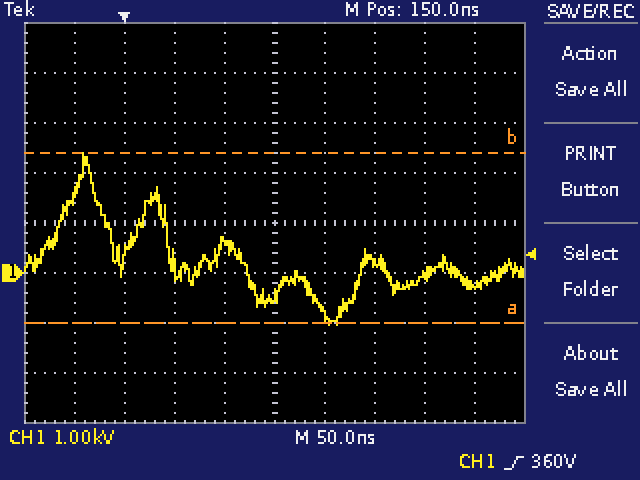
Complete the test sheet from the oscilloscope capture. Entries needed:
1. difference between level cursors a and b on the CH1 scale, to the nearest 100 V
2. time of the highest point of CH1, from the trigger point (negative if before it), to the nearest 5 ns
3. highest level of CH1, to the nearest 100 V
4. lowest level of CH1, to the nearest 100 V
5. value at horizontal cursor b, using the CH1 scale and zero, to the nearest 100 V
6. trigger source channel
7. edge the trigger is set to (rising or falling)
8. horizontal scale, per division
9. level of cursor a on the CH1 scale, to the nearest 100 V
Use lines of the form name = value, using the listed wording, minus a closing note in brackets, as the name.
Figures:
difference between level cursors a and b on the CH1 scale, to the nearest 100 V = 3.4 kV
time of the highest point of CH1, from the trigger point (negative if before it), to the nearest 5 ns = -40 ns
highest level of CH1, to the nearest 100 V = 2.4 kV
lowest level of CH1, to the nearest 100 V = -1.0 kV
value at horizontal cursor b, using the CH1 scale and zero, to the nearest 100 V = 2.4 kV
trigger source channel = CH1
edge the trigger is set to = rising
horizontal scale, per division = 50 ns
level of cursor a on the CH1 scale, to the nearest 100 V = -1.0 kV
